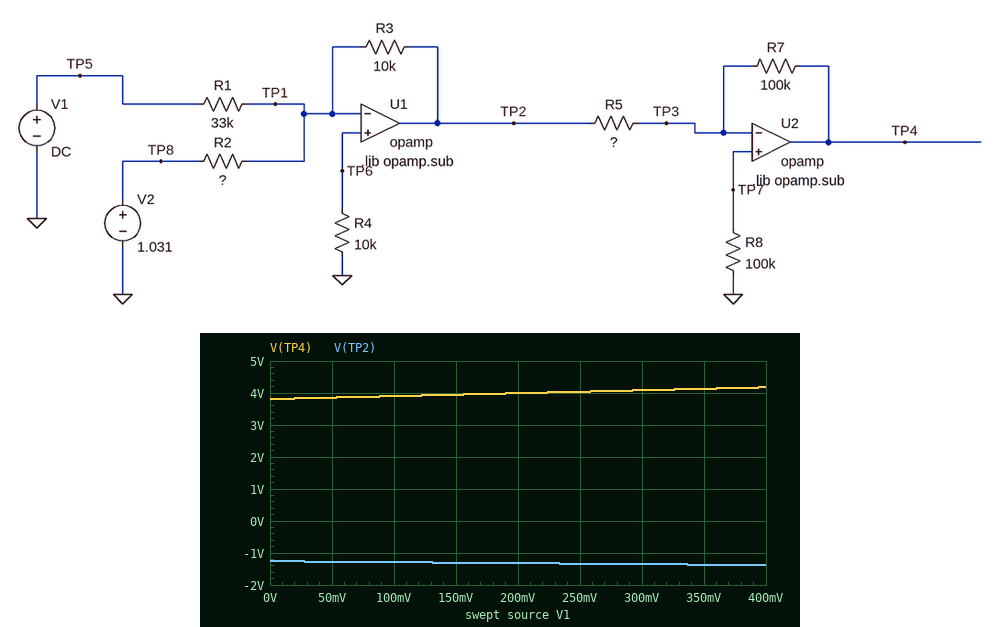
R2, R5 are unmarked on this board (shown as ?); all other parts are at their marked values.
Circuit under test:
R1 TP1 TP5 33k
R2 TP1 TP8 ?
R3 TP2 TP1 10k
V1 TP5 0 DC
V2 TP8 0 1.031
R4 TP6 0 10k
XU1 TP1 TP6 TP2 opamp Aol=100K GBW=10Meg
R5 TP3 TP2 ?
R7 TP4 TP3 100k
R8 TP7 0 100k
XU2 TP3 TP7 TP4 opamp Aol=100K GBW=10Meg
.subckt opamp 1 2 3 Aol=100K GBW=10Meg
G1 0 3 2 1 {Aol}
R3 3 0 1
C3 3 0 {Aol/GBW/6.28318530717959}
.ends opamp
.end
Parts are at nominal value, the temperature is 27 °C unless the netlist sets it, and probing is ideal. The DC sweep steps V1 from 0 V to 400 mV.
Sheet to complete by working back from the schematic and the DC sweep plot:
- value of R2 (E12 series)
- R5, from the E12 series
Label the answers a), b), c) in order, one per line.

a) 8.2 kΩ
b) 33 kΩ
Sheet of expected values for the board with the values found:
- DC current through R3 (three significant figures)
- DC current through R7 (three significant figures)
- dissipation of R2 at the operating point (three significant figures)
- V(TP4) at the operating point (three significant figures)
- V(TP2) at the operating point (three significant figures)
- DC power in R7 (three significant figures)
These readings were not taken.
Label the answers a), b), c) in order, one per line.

a) 126 µA
b) 38.1 µA
c) 130 µW
d) 3.81 V
e) -1.26 V
f) 145 µW
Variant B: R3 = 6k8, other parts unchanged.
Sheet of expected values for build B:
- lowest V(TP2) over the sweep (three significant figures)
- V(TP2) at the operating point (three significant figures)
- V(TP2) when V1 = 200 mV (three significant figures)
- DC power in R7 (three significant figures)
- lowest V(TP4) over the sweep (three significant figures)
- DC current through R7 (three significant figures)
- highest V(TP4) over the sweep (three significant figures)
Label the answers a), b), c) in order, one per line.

a) -937 mV
b) -855 mV
c) -896 mV
d) 67.1 µW
e) 2.59 V
f) 25.9 µA
g) 2.84 V
